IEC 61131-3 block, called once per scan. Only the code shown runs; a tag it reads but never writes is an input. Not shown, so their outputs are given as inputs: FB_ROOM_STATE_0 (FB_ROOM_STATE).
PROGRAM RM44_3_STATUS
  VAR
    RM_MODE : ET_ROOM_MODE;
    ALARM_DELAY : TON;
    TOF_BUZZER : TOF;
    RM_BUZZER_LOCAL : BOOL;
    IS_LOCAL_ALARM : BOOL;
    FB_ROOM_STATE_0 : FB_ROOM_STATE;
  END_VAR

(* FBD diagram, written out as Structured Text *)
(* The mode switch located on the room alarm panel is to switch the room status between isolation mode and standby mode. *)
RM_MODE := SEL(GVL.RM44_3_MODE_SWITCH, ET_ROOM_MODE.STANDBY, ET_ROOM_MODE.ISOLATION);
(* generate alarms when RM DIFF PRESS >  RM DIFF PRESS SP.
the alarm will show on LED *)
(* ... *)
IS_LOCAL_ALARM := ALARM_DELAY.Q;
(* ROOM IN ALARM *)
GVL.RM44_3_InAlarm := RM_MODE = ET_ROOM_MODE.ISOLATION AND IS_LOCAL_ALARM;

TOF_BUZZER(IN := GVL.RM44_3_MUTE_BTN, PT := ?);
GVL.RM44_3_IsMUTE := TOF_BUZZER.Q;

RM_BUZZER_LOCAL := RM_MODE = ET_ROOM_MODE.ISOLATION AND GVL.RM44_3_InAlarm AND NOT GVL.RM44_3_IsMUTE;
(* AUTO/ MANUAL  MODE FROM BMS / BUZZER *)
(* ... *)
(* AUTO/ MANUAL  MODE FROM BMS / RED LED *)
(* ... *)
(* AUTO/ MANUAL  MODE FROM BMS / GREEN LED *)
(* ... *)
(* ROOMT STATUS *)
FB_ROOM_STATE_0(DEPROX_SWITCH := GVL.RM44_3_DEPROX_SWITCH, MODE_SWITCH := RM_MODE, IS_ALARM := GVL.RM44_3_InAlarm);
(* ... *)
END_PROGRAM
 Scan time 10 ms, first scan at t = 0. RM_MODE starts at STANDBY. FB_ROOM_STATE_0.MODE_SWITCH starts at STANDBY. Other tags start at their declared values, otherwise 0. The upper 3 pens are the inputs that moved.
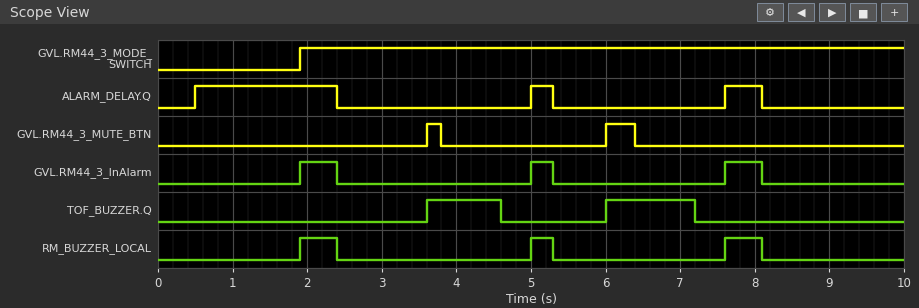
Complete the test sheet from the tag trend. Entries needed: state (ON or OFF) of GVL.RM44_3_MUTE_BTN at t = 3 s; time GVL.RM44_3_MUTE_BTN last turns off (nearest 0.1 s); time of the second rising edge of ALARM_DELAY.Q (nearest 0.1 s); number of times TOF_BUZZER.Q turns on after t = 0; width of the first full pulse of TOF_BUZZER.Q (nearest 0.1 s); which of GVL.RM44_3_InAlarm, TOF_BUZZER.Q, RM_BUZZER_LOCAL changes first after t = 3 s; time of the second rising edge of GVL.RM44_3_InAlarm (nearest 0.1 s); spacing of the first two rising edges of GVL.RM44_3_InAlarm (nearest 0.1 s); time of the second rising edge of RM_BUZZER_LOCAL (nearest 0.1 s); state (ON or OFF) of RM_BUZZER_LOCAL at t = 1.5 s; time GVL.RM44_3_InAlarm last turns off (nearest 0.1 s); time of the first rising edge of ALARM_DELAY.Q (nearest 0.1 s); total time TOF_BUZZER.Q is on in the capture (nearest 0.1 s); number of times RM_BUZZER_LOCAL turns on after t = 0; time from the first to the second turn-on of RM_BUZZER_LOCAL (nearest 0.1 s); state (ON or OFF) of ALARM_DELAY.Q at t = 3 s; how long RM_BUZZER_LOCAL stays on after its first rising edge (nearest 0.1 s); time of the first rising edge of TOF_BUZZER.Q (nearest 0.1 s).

OFF
6.4 s
5.0 s
2
1.0 s
TOF_BUZZER.Q
5.0 s
3.1 s
5.0 s
OFF
8.1 s
0.5 s
2.2 s
3
3.1 s
OFF
0.5 s
3.6 s
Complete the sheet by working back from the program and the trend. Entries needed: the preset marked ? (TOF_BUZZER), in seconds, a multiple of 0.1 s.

0.8 s
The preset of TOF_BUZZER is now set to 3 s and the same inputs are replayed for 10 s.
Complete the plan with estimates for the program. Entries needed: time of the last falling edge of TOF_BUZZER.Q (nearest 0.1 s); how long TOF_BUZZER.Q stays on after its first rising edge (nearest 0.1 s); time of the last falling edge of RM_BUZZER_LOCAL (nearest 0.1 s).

9.4 s
5.8 s
2.4 s
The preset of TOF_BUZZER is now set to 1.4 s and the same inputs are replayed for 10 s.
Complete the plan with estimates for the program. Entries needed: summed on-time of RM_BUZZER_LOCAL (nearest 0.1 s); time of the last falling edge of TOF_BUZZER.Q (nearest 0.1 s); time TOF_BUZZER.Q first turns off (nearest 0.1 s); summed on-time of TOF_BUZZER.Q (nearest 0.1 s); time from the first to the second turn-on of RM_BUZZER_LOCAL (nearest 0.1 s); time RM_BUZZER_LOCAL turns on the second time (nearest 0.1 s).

0.9 s
7.8 s
5.2 s
3.4 s
3.3 s
5.2 s
